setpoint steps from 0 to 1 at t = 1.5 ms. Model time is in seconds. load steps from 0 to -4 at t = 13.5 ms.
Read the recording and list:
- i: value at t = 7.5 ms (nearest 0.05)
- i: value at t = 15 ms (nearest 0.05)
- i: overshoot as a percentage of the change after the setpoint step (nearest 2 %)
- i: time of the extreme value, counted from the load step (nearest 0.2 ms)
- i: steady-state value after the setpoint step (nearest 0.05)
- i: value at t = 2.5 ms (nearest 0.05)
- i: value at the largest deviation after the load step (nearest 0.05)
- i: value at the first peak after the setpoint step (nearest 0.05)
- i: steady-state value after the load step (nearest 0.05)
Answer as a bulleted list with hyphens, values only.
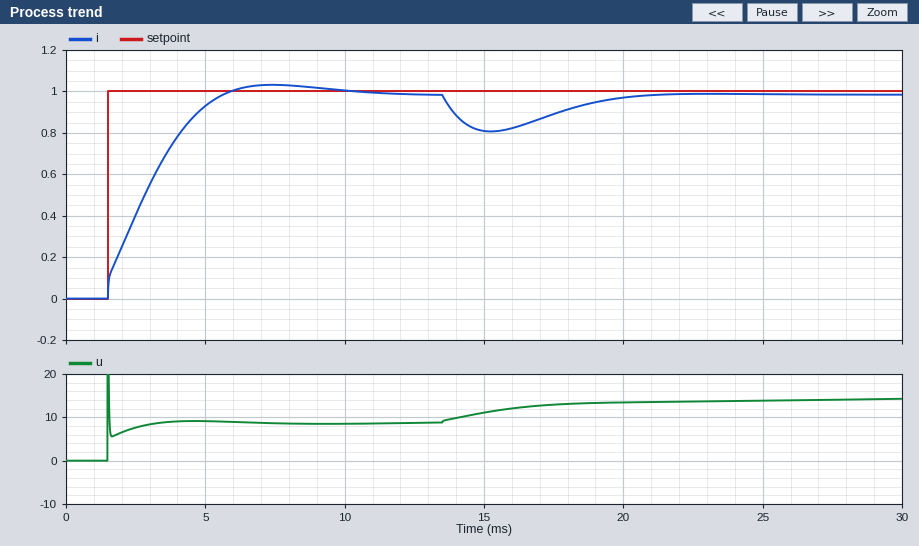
- 1.05
- 0.80
- 4 %
- 1.8 ms
- 1.00
- 0.40
- 0.80
- 1.05
- 1.00
